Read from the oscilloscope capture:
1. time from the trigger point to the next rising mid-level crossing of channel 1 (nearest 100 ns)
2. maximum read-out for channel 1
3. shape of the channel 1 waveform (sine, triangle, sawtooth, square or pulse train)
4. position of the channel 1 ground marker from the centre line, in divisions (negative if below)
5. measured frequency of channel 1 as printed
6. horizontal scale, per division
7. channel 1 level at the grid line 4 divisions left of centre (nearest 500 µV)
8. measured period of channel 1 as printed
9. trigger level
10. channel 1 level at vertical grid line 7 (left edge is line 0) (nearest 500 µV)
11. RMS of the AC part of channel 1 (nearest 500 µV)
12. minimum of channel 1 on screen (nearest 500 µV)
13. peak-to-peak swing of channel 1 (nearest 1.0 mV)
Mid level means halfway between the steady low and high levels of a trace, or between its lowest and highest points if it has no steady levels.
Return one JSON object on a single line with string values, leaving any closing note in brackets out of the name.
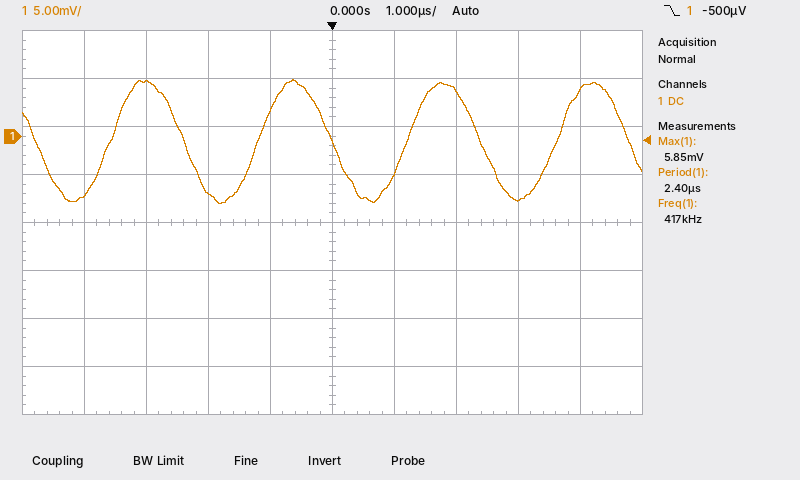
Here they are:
{"time from the trigger point to the next rising mid-level crossing of channel 1": "1.2 µs", "maximum read-out for channel 1": "5.85 mV", "shape of the channel 1 waveform": "sine", "position of the channel 1 ground marker from the centre line, in divisions": "+1.8 div", "measured frequency of channel 1 as printed": "417 kHz", "horizontal scale, per division": "1 µs", "channel 1 level at the grid line 4 divisions left of centre": "-6.0 mV", "measured period of channel 1 as printed": "2.40 µs", "trigger level": "-500 µV", "channel 1 level at vertical grid line 7 (left edge is line 0)": "4.5 mV", "RMS of the AC part of channel 1": "4.5 mV", "minimum of channel 1 on screen": "-7.0 mV", "peak-to-peak swing of channel 1": "13.0 mV"}
